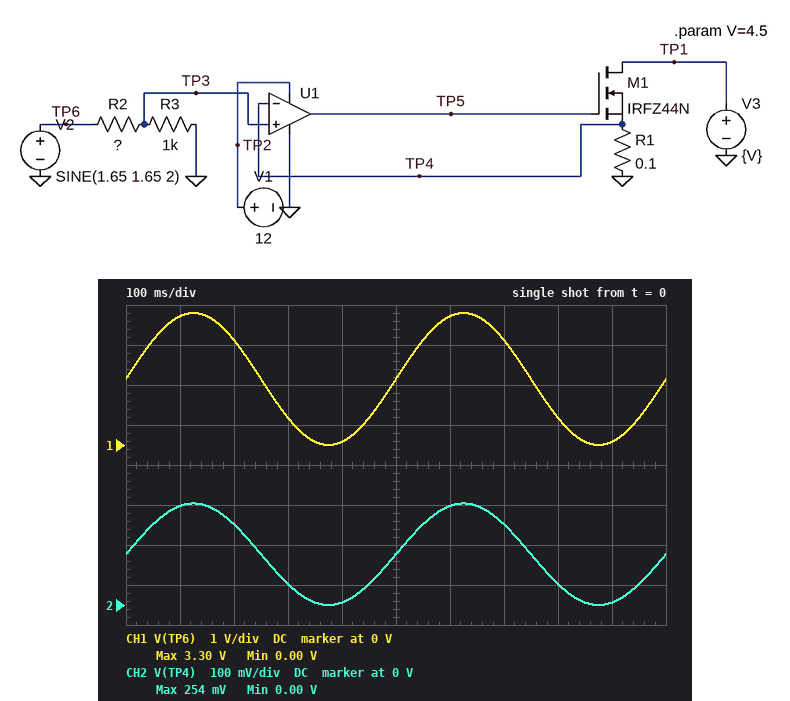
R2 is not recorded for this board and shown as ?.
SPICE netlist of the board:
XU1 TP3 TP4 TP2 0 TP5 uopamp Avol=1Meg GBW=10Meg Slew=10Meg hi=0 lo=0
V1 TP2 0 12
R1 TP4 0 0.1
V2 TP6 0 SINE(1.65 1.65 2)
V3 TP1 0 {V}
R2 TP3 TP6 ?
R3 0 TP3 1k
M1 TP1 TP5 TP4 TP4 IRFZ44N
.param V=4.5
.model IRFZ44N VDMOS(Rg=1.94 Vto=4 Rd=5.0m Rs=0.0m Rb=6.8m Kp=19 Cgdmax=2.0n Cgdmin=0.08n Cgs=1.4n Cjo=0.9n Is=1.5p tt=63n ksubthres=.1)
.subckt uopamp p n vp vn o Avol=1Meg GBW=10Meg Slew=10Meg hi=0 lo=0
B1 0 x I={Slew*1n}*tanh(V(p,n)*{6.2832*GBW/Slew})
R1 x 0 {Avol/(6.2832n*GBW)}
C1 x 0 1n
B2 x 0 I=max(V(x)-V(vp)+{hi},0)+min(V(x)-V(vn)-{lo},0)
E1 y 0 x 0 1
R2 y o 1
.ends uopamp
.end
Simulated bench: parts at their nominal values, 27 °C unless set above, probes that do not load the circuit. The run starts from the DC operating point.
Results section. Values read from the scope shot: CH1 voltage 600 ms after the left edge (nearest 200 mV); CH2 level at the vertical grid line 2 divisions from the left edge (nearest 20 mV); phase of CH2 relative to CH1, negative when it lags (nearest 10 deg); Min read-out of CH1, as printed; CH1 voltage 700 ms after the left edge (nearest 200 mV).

3.2 V
200 mV
0 deg
0.00 V
2.6 V
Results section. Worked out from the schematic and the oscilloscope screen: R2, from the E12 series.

12 kΩ
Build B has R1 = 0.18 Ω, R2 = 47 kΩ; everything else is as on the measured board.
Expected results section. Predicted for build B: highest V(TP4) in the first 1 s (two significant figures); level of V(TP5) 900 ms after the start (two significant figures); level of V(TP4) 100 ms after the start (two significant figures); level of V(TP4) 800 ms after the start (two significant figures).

69 mV
3.9 V
67 mV
14 mV
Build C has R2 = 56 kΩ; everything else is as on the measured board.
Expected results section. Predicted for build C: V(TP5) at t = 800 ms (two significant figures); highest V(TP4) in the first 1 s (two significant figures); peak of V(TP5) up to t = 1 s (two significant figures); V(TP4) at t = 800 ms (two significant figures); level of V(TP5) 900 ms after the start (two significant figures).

4.1 V
58 mV
4.3 V
12 mV
3.9 V
